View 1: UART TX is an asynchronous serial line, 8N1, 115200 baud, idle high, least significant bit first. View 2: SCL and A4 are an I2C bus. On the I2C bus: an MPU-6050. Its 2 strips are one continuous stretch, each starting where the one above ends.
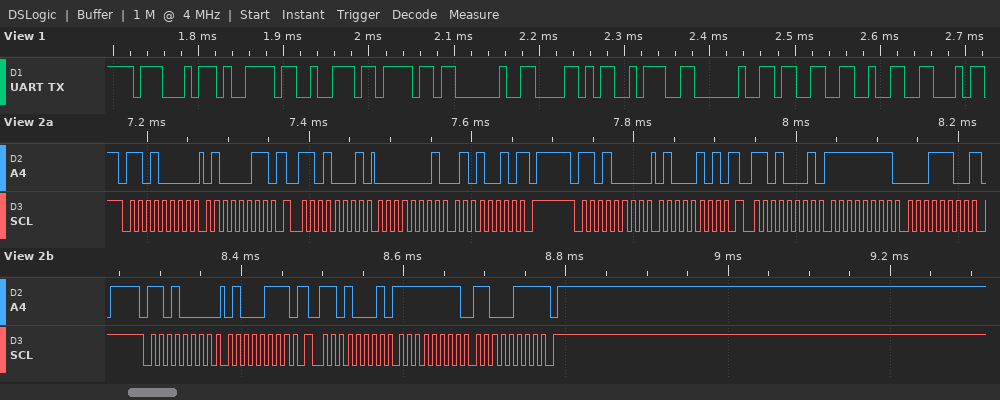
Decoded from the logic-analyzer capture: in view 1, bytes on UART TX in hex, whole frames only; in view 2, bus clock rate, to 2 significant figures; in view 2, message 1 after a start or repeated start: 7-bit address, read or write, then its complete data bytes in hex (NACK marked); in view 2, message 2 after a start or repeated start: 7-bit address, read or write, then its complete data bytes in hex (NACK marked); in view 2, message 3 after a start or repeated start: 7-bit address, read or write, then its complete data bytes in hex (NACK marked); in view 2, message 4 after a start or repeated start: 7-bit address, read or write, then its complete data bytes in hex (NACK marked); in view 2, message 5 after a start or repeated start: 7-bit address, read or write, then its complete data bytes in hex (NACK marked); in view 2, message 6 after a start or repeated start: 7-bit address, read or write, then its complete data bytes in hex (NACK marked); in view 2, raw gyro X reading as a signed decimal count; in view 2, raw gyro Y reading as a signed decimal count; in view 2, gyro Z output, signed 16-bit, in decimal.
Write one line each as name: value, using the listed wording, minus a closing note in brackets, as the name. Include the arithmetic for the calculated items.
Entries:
in view 1, bytes on UART TX in hex, whole frames only: 47 79 72 6F 20 58 3A 20 33 32
in view 2, bus clock rate, to 2 significant figures: 100 kHz
in view 2, message 1 after a start or repeated start: 7-bit address, read or write, then its complete data bytes in hex: 0x68 write: 43
in view 2, message 2 after a start or repeated start: 7-bit address, read or write, then its complete data bytes in hex: 0x68 read: 01 52 NACK
in view 2, message 3 after a start or repeated start: 7-bit address, read or write, then its complete data bytes in hex: 0x68 write: 45
in view 2, message 4 after a start or repeated start: 7-bit address, read or write, then its complete data bytes in hex: 0x68 read: FF 1C NACK
in view 2, message 5 after a start or repeated start: 7-bit address, read or write, then its complete data bytes in hex: 0x68 write: 47
in view 2, message 6 after a start or repeated start: 7-bit address, read or write, then its complete data bytes in hex: 0x68 read: FF C7 NACK
in view 2, raw gyro X reading as a signed decimal count: 0x0152 = 338
in view 2, raw gyro Y reading as a signed decimal count: 0xFF1C = -228
in view 2, gyro Z output, signed 16-bit, in decimal: 0xFFC7 = -57
